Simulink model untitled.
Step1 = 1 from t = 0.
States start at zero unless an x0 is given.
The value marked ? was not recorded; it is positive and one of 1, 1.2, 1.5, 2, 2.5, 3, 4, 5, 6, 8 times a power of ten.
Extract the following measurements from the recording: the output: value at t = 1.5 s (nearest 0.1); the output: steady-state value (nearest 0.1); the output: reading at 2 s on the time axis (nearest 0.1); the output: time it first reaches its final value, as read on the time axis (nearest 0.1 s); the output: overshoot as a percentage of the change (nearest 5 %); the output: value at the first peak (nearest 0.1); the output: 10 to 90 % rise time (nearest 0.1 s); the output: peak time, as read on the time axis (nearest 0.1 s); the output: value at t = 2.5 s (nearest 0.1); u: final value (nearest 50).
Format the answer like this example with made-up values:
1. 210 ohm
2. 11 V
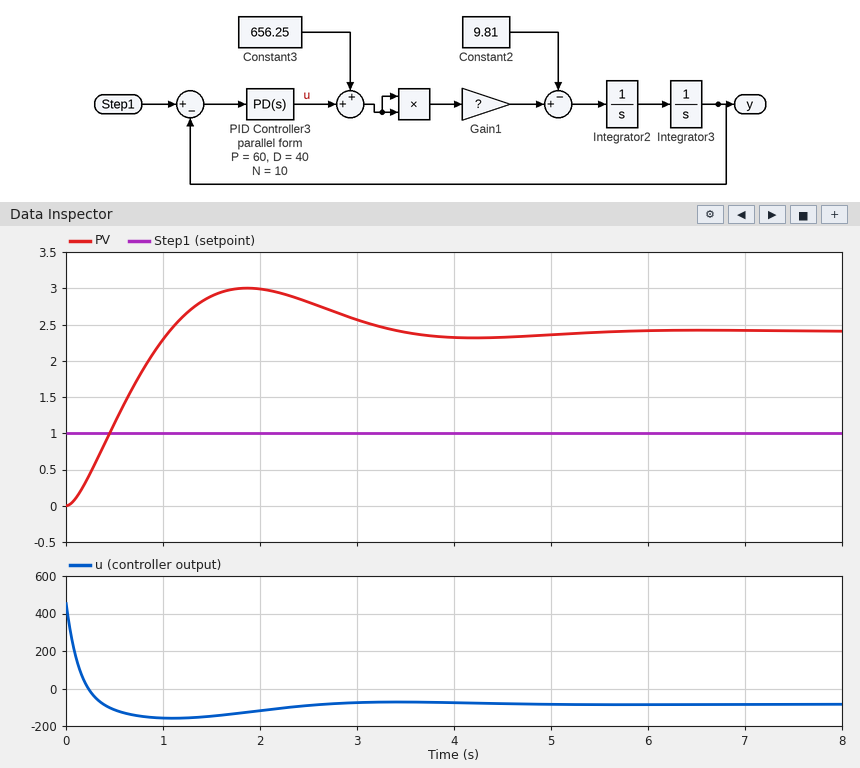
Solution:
1. 2.9
2. 2.4
3. 3.0
4. 1.1 s
5. 25 %
6. 3.0
7. 0.8 s
8. 1.9 s
9. 2.8
10. -100
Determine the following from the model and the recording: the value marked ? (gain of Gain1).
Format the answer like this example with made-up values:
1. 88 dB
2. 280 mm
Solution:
1. 3e-05
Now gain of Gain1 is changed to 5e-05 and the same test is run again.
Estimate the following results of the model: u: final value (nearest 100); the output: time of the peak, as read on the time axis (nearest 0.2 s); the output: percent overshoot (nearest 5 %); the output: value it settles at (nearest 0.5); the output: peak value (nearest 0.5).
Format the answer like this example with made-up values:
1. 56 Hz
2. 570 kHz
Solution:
1. -200
2. 1.8 s
3. 20 %
4. 4.5
5. 5.5
